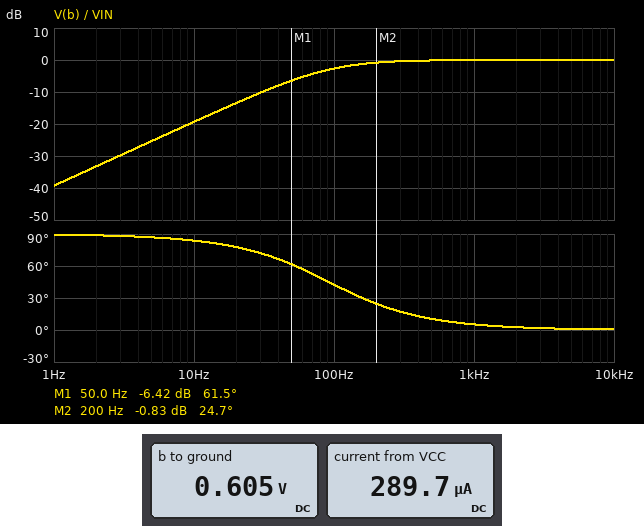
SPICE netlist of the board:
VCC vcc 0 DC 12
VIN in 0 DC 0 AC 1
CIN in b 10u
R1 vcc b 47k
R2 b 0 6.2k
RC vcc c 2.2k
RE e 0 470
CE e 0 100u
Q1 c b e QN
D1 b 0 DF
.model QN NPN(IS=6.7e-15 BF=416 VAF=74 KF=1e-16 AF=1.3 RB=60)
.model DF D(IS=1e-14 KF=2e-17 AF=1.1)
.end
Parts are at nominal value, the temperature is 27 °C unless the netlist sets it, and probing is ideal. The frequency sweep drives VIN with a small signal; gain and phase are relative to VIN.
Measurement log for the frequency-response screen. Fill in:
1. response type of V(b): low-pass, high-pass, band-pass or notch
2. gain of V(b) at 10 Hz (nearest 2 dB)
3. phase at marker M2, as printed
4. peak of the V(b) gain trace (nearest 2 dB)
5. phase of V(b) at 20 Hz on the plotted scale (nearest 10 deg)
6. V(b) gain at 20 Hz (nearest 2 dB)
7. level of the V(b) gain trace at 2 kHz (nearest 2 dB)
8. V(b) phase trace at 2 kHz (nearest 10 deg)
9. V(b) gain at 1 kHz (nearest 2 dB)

high-pass
-20 dB
24.7 deg
0 dB
80 deg
-14 dB
0 dB
0 deg
0 dB
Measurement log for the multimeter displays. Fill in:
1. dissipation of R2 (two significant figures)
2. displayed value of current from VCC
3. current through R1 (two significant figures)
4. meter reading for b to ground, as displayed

59 µW
289.7 µA
240 µA
0.605 V
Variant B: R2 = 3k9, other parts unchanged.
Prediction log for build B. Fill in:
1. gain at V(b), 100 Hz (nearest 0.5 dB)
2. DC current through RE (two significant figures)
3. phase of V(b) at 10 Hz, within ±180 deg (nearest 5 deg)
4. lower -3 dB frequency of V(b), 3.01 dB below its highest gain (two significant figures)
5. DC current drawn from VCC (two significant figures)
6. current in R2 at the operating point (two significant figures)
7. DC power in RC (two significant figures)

-1.5 dB
36 µA
80 deg
60 Hz
280 µA
150 µA
2.9 µW
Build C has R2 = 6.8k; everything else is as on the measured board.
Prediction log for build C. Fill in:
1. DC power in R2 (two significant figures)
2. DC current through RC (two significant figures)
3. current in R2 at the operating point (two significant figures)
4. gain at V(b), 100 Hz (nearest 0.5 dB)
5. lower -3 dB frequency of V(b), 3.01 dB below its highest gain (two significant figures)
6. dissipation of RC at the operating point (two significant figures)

54 µW
49 µA
89 µA
-3.0 dB
97 Hz
5.2 µW
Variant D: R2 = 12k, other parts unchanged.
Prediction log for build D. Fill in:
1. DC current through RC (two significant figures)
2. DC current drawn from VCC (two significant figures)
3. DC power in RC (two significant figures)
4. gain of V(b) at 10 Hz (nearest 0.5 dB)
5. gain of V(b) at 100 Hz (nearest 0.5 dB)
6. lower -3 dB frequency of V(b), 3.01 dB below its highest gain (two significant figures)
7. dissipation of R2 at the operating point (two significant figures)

55 µA
300 µA
6.6 µW
-21.5 dB
-4.0 dB
120 Hz
31 µW
